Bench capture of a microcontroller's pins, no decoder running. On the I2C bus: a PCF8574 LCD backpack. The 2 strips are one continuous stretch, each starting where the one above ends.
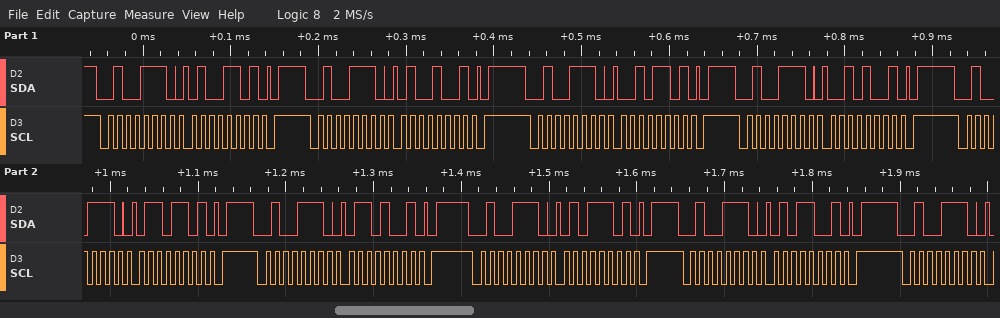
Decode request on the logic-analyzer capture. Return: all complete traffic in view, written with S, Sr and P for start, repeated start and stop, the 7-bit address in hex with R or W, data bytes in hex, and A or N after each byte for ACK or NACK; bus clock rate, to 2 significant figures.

S 27W A 4D A P S 27W A 49 A P S 27W A 2D A P S 27W A 29 A P S 27W A 6D A P S 27W A 69 A P S 27W A 5D A P S 27W A 59 A P S 27W A
100 kHz
